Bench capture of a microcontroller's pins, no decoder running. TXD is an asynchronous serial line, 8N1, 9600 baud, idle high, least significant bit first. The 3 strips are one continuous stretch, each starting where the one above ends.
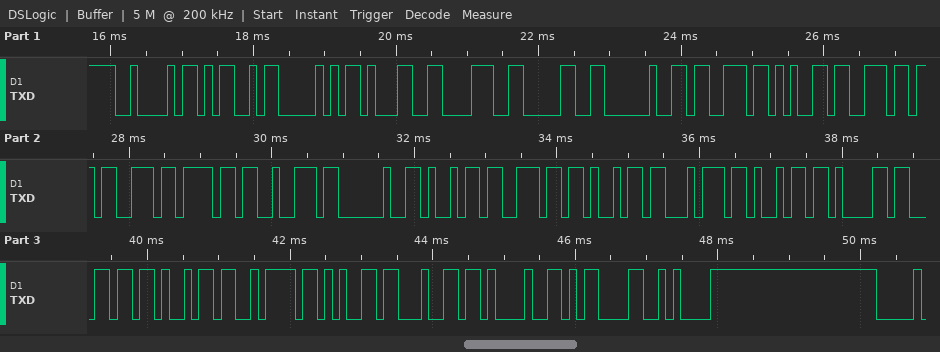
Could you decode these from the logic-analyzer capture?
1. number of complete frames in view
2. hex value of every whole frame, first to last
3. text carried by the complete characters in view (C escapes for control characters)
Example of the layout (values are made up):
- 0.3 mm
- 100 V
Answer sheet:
- 28
- 42 4D 50 31 38 30 20 73 65 6E 73 6F 72 20 69 6E 69 74 69 61 6C 69 7A 65 64 21 0D 0A
- "BMP180 sensor initialized!\r\n"
